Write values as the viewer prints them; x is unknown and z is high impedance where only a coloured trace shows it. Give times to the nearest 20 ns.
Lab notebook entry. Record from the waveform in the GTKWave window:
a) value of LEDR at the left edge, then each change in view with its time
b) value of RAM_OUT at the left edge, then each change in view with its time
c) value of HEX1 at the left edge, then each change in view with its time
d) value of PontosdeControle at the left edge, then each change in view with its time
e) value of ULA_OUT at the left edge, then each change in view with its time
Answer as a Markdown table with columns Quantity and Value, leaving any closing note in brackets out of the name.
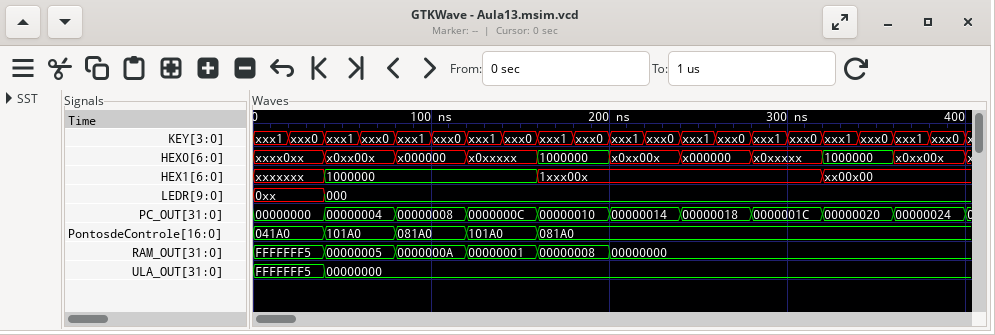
| Quantity | Value |
|---|---|
| value of LEDR at the left edge, then each change in view with its time | 0xx, 000 at 40 ns |
| value of RAM_OUT at the left edge, then each change in view with its time | FFFFFFF5, 00000005 at 40 ns, 0000000A at 80 ns, 00000001 at 120 ns, 00000008 at 160 ns, 00000000 at 200 ns |
| value of HEX1 at the left edge, then each change in view with its time | xxxxxxx, 1000000 at 40 ns, 1xxx00x at 160 ns, xx00x00 at 320 ns |
| value of PontosdeControle at the left edge, then each change in view with its time | 041A0, 101A0 at 40 ns, 081A0 at 80 ns, 101A0 at 120 ns, 081A0 at 160 ns |
| value of ULA_OUT at the left edge, then each change in view with its time | FFFFFFF5, 00000000 at 40 ns |
